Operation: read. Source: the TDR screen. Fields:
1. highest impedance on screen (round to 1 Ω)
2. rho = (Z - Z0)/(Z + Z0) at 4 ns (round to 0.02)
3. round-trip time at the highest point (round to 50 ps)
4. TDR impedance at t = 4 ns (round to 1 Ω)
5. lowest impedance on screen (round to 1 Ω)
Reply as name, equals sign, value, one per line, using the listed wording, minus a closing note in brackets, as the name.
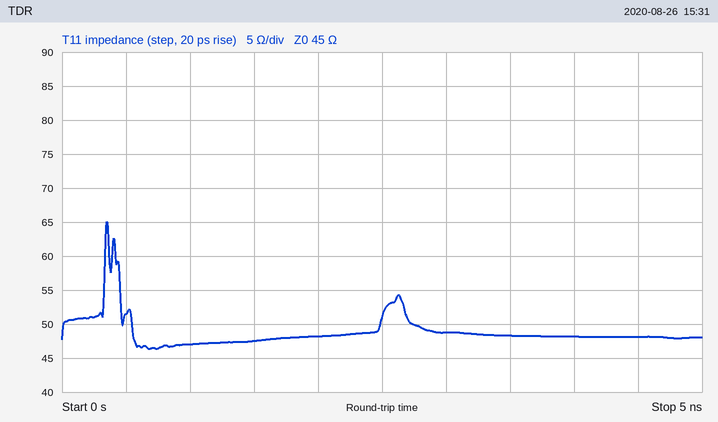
highest impedance on screen = 65 Ω
rho = (Z - Z0)/(Z + Z0) at 4 ns = +0.04
round-trip time at the highest point = 350 ps
TDR impedance at t = 4 ns = 48 Ω
lowest impedance on screen = 46 Ω
